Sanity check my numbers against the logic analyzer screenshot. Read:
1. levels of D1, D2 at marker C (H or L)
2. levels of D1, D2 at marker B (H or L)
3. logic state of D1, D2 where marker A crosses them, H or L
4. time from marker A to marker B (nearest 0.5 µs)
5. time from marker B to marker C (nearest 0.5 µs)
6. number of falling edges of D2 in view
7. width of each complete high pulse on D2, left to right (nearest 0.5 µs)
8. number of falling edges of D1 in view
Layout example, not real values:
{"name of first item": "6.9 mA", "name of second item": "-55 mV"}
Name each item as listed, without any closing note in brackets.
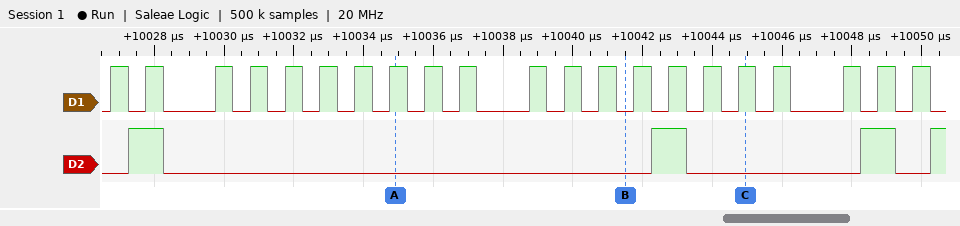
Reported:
{"levels of D1, D2 at marker C": "D1=H, D2=L", "levels of D1, D2 at marker B": "D1=L, D2=L", "logic state of D1, D2 where marker A crosses them, H or L": "D1=H, D2=L", "time from marker A to marker B": "6.5 µs", "time from marker B to marker C": "3.5 µs", "number of falling edges of D2 in view": "3", "width of each complete high pulse on D2, left to right": "1 µs, 1 µs, 1 µs", "number of falling edges of D1 in view": "21"}
